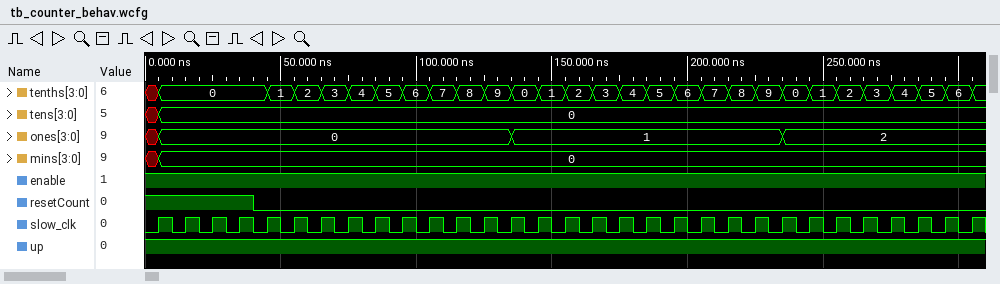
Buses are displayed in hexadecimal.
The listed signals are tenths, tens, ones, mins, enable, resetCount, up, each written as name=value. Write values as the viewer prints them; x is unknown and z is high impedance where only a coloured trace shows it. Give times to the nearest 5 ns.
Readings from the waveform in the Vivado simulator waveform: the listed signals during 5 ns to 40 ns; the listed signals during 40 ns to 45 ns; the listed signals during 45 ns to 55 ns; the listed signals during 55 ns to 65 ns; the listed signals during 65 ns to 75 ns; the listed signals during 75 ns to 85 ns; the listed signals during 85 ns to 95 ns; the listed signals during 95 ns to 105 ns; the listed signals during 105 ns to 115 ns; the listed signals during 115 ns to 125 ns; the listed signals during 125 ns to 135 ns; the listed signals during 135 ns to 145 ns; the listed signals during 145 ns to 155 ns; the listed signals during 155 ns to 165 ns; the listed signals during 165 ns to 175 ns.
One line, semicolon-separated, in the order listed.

tenths=0, tens=0, ones=0, mins=0, enable=1, resetCount=1, up=1; tenths=0, tens=0, ones=0, mins=0, enable=1, resetCount=0, up=1; tenths=1, tens=0, ones=0, mins=0, enable=1, resetCount=0, up=1; tenths=2, tens=0, ones=0, mins=0, enable=1, resetCount=0, up=1; tenths=3, tens=0, ones=0, mins=0, enable=1, resetCount=0, up=1; tenths=4, tens=0, ones=0, mins=0, enable=1, resetCount=0, up=1; tenths=5, tens=0, ones=0, mins=0, enable=1, resetCount=0, up=1; tenths=6, tens=0, ones=0, mins=0, enable=1, resetCount=0, up=1; tenths=7, tens=0, ones=0, mins=0, enable=1, resetCount=0, up=1; tenths=8, tens=0, ones=0, mins=0, enable=1, resetCount=0, up=1; tenths=9, tens=0, ones=0, mins=0, enable=1, resetCount=0, up=1; tenths=0, tens=0, ones=1, mins=0, enable=1, resetCount=0, up=1; tenths=1, tens=0, ones=1, mins=0, enable=1, resetCount=0, up=1; tenths=2, tens=0, ones=1, mins=0, enable=1, resetCount=0, up=1; tenths=3, tens=0, ones=1, mins=0, enable=1, resetCount=0, up=1
